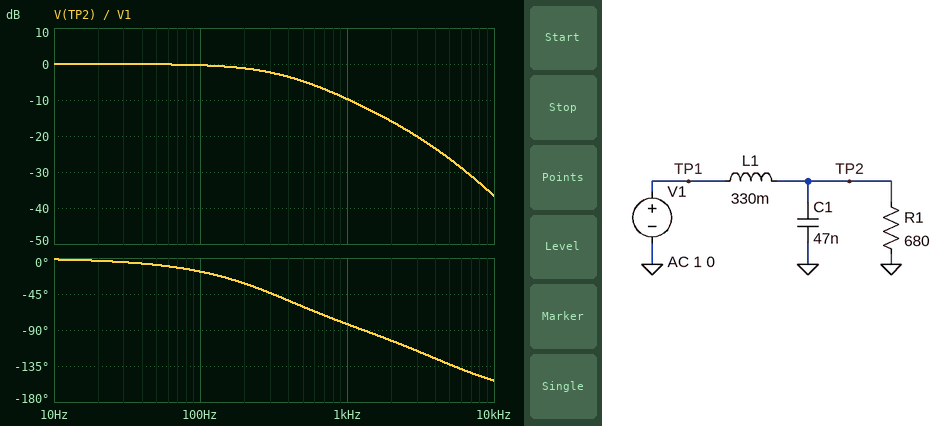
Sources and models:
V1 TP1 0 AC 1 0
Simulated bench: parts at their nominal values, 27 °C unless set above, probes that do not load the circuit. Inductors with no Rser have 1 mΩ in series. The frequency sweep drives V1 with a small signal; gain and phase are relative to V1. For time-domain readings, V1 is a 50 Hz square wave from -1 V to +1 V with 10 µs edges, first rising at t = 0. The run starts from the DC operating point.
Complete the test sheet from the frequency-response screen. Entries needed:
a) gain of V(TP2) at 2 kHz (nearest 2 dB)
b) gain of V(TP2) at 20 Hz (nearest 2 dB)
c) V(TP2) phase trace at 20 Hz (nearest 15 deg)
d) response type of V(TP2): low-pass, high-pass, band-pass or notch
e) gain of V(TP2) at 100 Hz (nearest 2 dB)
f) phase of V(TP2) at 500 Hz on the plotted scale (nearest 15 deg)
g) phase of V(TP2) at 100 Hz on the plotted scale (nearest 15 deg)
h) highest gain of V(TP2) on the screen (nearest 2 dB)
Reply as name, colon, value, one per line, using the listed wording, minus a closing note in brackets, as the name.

gain of V(TP2) at 2 kHz: -16 dB
gain of V(TP2) at 20 Hz: 0 dB
V(TP2) phase trace at 20 Hz: 0 deg
response type of V(TP2): low-pass, high-pass, band-pass or notch: low-pass
gain of V(TP2) at 100 Hz: 0 dB
phase of V(TP2) at 500 Hz on the plotted scale: -60 deg
phase of V(TP2) at 100 Hz on the plotted scale: -15 deg
highest gain of V(TP2) on the screen: 0 dB
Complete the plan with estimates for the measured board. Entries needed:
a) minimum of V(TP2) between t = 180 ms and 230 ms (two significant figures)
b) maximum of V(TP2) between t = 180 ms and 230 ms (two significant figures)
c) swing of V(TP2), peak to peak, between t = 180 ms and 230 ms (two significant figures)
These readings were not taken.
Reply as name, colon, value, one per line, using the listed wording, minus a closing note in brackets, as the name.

minimum of V(TP2) between t = 180 ms and 230 ms: -1.0 V
maximum of V(TP2) between t = 180 ms and 230 ms: 1.0 V
swing of V(TP2), peak to peak, between t = 180 ms and 230 ms: 2.0 V
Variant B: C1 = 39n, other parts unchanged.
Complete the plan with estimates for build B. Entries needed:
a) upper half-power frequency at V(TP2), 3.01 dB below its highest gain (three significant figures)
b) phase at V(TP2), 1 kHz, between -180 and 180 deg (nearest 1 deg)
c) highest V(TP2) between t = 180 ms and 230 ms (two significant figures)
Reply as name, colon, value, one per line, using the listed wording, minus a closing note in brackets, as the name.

upper half-power frequency at V(TP2), 3.01 dB below its highest gain: 347 Hz
phase at V(TP2), 1 kHz, between -180 and 180 deg: -81 deg
highest V(TP2) between t = 180 ms and 230 ms: 1.0 V
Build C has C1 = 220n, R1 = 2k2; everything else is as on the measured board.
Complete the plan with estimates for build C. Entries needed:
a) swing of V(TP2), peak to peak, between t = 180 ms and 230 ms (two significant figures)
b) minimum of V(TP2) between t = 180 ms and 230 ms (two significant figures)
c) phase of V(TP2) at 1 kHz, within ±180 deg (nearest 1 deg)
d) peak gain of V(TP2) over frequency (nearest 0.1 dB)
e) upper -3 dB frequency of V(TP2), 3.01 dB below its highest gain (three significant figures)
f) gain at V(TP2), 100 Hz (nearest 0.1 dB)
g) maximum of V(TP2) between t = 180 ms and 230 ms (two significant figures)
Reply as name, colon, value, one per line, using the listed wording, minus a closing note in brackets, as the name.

swing of V(TP2), peak to peak, between t = 180 ms and 230 ms: 3.6 V
minimum of V(TP2) between t = 180 ms and 230 ms: -1.8 V
phase of V(TP2) at 1 kHz, within ±180 deg: -153 deg
peak gain of V(TP2) over frequency: 5.4 dB
upper -3 dB frequency of V(TP2), 3.01 dB below its highest gain: 694 Hz
gain at V(TP2), 100 Hz: 0.2 dB
maximum of V(TP2) between t = 180 ms and 230 ms: 1.8 V
